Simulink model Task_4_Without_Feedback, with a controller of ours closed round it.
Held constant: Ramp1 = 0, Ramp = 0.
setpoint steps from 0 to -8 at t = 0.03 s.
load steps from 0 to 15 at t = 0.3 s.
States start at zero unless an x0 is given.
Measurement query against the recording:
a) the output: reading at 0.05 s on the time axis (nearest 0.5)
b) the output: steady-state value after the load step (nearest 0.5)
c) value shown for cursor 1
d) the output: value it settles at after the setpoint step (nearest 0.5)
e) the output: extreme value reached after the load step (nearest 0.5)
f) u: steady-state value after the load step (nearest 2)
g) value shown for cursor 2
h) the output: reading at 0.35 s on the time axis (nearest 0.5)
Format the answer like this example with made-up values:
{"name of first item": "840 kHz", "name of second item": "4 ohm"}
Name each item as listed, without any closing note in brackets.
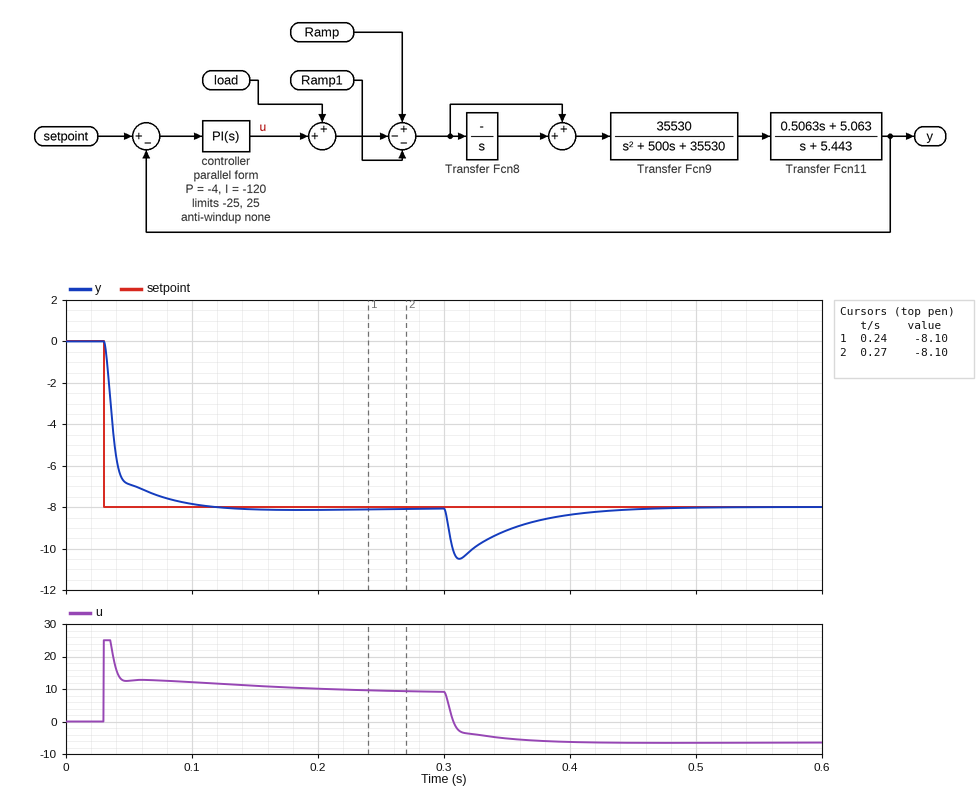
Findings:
{"the output: reading at 0.05 s on the time axis": "-7.0", "the output: steady-state value after the load step": "-8.0", "value shown for cursor 1": "-8.10", "the output: value it settles at after the setpoint step": "-8.0", "the output: extreme value reached after the load step": "-10.5", "u: steady-state value after the load step": "-6", "value shown for cursor 2": "-8.10", "the output: reading at 0.35 s on the time axis": "-9.0"}
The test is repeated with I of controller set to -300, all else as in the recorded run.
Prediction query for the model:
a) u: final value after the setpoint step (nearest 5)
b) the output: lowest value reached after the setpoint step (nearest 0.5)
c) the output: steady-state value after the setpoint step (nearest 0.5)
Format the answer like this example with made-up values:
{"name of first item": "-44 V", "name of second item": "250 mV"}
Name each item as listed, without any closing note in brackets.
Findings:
{"u: final value after the setpoint step": "10", "the output: lowest value reached after the setpoint step": "-8.5", "the output: steady-state value after the setpoint step": "-8.0"}
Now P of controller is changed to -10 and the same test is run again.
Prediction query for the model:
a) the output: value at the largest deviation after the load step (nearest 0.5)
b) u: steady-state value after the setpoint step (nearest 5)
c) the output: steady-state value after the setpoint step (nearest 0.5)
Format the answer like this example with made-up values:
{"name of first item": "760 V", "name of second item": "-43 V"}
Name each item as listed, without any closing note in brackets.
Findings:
{"the output: value at the largest deviation after the load step": "-9.5", "u: steady-state value after the setpoint step": "10", "the output: steady-state value after the setpoint step": "-8.0"}
